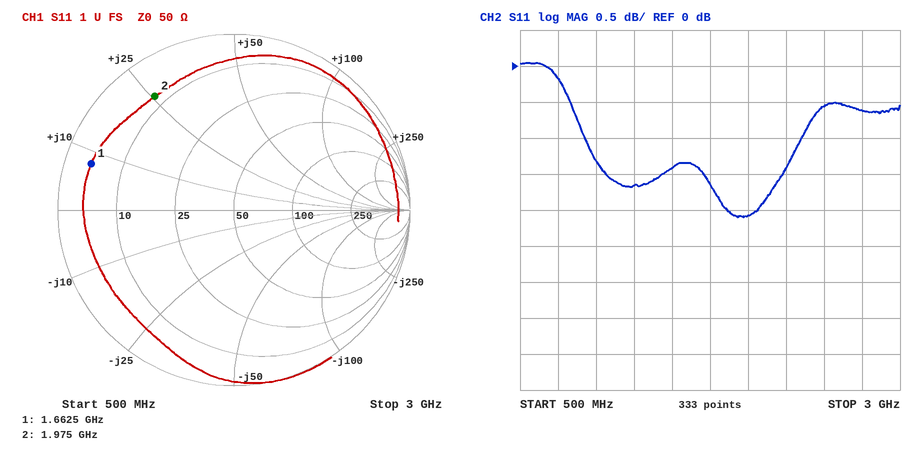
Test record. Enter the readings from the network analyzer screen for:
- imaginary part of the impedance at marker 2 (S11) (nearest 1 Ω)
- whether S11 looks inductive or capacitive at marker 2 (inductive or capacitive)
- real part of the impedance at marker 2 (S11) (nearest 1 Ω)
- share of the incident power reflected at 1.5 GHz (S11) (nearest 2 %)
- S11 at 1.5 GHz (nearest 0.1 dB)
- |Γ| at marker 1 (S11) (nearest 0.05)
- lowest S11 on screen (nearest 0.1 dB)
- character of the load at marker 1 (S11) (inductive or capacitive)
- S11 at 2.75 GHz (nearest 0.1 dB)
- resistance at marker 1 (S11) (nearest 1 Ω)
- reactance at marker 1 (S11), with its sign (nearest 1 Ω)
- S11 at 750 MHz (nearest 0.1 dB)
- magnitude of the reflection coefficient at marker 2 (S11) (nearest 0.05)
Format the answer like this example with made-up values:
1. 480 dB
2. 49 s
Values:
1. +26 Ω
2. inductive
3. 8 Ω
4. 72 %
5. -1.4 dB
6. 0.85
7. -2.1 dB
8. inductive
9. -0.6 dB
10. 4 Ω
11. +8 Ω
12. -0.2 dB
13. 0.80
